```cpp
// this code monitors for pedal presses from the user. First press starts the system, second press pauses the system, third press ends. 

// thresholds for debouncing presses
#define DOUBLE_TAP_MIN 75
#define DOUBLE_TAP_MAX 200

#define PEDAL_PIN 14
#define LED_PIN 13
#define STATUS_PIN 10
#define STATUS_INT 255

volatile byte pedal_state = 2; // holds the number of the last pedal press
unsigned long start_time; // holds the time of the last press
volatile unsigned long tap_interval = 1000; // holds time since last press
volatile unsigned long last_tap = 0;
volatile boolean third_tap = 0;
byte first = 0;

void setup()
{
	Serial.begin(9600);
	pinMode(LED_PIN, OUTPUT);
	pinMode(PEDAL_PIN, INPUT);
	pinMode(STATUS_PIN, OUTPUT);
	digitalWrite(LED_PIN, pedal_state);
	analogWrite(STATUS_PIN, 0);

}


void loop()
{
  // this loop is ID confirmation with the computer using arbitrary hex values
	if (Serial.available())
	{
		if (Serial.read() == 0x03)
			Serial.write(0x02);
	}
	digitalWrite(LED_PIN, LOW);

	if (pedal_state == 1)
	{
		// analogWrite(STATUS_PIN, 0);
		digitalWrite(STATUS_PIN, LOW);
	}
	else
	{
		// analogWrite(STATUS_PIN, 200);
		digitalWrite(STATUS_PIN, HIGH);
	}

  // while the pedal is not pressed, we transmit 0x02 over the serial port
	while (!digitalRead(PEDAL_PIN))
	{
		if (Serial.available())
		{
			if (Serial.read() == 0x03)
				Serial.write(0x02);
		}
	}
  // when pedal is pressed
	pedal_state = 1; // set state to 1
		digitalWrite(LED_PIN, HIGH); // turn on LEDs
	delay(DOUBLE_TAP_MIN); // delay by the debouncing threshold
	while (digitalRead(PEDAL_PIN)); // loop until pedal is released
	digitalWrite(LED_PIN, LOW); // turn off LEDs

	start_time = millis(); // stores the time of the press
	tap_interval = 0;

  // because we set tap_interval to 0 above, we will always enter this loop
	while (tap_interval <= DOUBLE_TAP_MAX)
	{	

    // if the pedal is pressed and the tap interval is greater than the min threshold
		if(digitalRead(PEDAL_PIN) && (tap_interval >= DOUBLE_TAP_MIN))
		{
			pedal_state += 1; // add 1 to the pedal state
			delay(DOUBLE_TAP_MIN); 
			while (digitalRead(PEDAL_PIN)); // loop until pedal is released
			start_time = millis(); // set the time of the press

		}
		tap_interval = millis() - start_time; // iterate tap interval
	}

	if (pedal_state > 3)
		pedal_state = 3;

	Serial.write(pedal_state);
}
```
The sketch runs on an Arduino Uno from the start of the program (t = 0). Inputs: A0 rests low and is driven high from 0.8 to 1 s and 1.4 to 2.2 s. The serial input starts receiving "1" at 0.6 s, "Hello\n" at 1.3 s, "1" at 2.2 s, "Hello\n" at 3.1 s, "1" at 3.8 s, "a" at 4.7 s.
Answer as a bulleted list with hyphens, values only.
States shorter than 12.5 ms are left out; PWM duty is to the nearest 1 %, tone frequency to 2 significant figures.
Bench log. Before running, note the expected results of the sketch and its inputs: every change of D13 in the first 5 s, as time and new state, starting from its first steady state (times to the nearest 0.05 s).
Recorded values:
- 0 s low; 0.8 s high; 1 s low; 1.4 s high; 2.2 s low
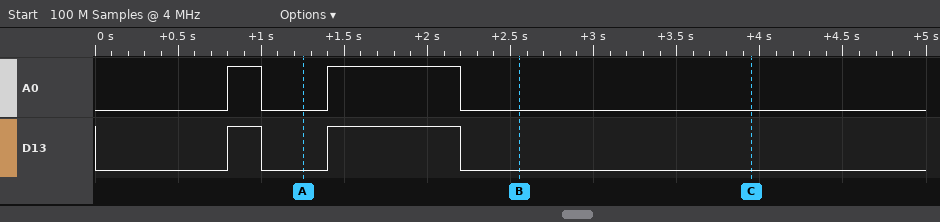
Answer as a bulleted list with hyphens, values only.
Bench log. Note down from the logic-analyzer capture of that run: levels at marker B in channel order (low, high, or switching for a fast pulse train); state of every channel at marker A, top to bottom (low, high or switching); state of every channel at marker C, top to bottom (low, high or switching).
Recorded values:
- A0 low, D13 low
- A0 low, D13 low
- A0 low, D13 low
